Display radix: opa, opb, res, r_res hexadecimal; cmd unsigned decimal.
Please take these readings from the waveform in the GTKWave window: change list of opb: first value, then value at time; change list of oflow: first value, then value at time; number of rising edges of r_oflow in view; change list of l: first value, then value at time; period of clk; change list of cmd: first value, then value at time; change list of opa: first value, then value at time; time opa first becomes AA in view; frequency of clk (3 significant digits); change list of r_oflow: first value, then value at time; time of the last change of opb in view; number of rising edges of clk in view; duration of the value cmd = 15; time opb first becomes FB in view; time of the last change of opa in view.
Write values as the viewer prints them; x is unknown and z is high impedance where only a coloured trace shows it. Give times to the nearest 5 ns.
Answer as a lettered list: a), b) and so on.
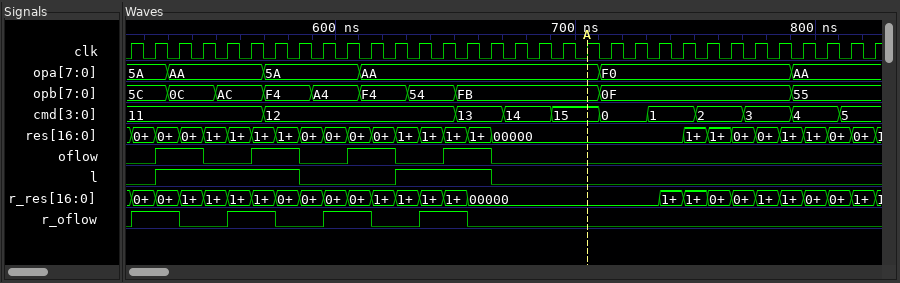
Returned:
a) 5C, 0C at 530 ns, AC at 550 ns, F4 at 570 ns, A4 at 590 ns, F4 at 610 ns, 54 at 630 ns, FB at 650 ns, 0F at 710 ns, 55 at 790 ns
b) 0, 1 at 525 ns, 0 at 545 ns, 1 at 565 ns, 0 at 585 ns, 1 at 605 ns, 0 at 625 ns, 1 at 645 ns, 0 at 665 ns
c) 4
d) 0, 1 at 525 ns, 0 at 585 ns, 1 at 625 ns, 0 at 665 ns
e) 10 ns
f) 11, 12 at 570 ns, 13 at 650 ns, 14 at 670 ns, 15 at 690 ns, 0 at 710 ns, 1 at 730 ns, 2 at 750 ns, 3 at 770 ns, 4 at 790 ns, 5 at 810 ns
g) 5A, AA at 530 ns, 5A at 570 ns, AA at 610 ns, F0 at 710 ns, AA at 790 ns
h) 530 ns
i) 100 MHz
j) 0, 1 at 515 ns, 0 at 535 ns, 1 at 555 ns, 0 at 575 ns, 1 at 595 ns, 0 at 615 ns, 1 at 635 ns, 0 at 655 ns
k) 790 ns
l) 32
m) 20 ns
n) 650 ns
o) 790 ns
